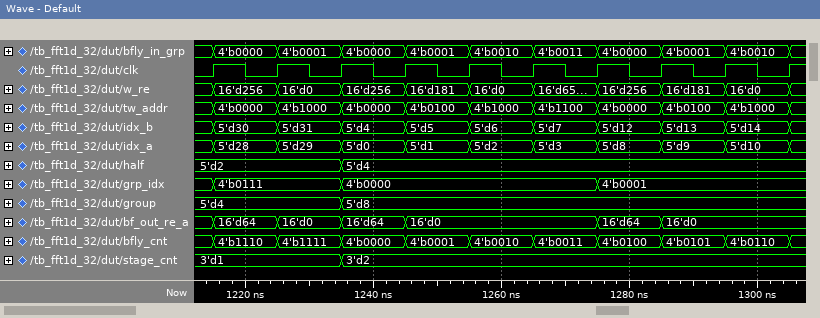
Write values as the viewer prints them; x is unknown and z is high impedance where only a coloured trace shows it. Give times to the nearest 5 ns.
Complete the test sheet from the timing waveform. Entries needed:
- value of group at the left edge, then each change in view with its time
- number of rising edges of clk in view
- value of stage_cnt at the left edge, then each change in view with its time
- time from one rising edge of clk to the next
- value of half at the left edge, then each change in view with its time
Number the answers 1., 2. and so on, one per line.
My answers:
1. 5'd4, 5'd8 at 1235 ns
2. 10
3. 3'd1, 3'd2 at 1235 ns
4. 10 ns
5. 5'd2, 5'd4 at 1235 ns
